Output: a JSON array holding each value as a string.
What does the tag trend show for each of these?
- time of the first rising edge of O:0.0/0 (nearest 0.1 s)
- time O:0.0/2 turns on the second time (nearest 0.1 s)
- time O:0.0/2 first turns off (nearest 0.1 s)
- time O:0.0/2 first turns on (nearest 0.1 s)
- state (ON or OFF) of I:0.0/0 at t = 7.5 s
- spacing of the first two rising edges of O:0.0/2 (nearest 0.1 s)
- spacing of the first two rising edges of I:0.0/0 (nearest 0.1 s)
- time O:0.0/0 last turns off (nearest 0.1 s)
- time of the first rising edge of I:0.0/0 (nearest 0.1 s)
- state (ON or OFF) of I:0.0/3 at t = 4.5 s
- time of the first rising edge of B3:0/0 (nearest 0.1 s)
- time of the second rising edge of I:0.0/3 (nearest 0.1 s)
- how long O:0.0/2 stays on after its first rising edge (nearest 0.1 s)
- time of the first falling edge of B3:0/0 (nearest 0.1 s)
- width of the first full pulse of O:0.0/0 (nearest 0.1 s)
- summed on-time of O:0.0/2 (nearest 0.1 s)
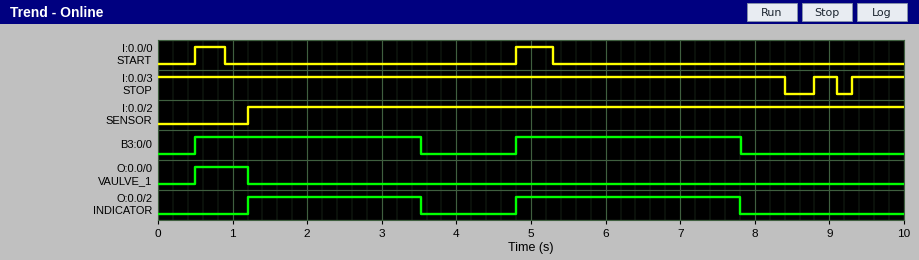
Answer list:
["0.5 s", "4.8 s", "3.5 s", "1.2 s", "OFF", "3.6 s", "4.3 s", "1.2 s", "0.5 s", "ON", "0.5 s", "9.3 s", "2.3 s", "3.5 s", "0.7 s", "5.3 s"]
